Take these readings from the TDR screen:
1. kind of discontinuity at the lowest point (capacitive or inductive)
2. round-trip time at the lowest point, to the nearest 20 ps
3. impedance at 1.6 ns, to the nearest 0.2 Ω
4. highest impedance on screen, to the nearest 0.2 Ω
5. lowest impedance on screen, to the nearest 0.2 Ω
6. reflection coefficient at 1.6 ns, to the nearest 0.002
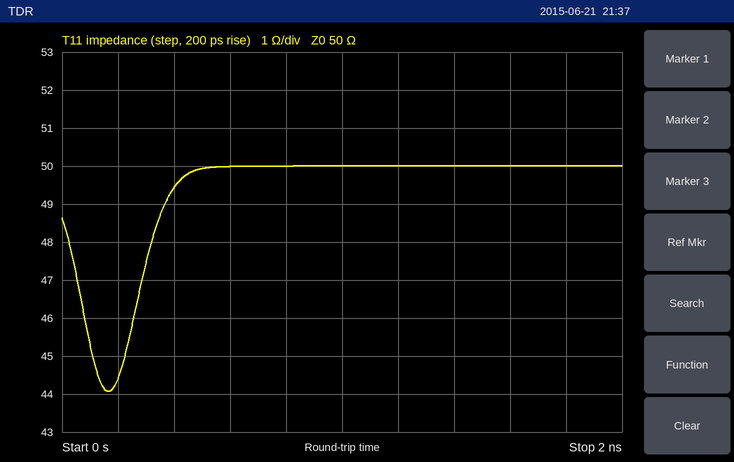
capacitive
160 ps
50.0 Ω
50.0 Ω
44.0 Ω
0.000
